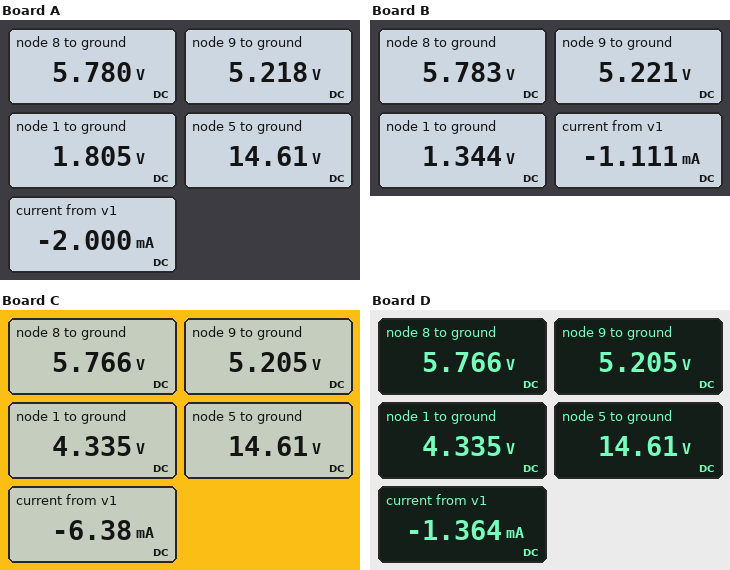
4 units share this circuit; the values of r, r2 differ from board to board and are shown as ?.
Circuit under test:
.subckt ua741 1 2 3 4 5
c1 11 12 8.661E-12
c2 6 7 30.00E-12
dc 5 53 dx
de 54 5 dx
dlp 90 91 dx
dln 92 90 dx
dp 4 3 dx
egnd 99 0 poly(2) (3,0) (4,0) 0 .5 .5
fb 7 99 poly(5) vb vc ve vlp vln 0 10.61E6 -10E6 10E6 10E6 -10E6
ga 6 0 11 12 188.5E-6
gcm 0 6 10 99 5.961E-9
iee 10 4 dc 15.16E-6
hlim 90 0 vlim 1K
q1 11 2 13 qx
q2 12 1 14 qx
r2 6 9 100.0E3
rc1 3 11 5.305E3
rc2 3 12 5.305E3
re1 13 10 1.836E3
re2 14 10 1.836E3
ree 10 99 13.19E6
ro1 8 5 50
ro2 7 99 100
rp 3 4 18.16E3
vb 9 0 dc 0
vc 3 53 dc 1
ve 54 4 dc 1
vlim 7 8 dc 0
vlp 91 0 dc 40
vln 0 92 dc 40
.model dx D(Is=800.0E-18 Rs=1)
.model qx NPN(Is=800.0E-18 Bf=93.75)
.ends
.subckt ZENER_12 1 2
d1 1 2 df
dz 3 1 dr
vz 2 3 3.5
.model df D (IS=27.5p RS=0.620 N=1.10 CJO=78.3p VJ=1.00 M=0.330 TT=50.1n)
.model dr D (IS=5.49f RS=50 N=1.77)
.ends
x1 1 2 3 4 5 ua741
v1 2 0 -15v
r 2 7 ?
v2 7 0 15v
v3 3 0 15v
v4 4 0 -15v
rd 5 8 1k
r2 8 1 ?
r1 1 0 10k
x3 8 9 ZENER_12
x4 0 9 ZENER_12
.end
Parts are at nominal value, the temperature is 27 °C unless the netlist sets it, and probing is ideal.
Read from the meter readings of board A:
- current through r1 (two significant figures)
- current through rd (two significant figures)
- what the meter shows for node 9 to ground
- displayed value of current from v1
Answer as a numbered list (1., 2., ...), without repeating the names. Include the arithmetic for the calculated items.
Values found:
1. (1.805 V) / 10 kΩ = 180 µA
2. (14.61 V - 5.78 V) / 1 kΩ = 8.8 mA
3. 5.218 V
4. -2.000 mA
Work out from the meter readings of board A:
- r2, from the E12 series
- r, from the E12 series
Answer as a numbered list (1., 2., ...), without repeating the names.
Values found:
1. 22 kΩ
2. 15 kΩ
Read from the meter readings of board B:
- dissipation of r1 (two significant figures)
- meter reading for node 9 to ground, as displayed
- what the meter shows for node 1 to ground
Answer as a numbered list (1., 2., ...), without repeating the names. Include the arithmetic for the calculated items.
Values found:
1. (1.344 V)^2 / 10 kΩ = 180 µW
2. 5.221 V
3. 1.344 V
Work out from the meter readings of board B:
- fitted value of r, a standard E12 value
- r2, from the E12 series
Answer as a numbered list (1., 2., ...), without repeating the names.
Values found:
1. 27 kΩ
2. 33 kΩ
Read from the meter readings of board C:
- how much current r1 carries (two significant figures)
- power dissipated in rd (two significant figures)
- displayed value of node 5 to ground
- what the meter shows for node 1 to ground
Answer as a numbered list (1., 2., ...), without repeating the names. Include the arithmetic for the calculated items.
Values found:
1. (4.335 V) / 10 kΩ = 430 µA
2. (14.61 V - 5.766 V)^2 / 1 kΩ = 78 mW
3. 14.61 V
4. 4.335 V
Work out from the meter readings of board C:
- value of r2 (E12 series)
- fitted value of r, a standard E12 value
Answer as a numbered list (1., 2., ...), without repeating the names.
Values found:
1. 3.3 kΩ
2. 4.7 kΩ
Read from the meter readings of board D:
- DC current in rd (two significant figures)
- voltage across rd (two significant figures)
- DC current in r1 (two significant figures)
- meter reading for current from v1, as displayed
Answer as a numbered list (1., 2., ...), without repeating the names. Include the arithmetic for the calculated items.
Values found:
1. (14.61 V - 5.766 V) / 1 kΩ = 8.8 mA
2. 14.61 V - 5.766 V = 8.8 V
3. (4.335 V) / 10 kΩ = 430 µA
4. -1.364 mA
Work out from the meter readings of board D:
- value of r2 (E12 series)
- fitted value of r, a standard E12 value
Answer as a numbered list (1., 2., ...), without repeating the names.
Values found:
1. 3.3 kΩ
2. 22 kΩ
